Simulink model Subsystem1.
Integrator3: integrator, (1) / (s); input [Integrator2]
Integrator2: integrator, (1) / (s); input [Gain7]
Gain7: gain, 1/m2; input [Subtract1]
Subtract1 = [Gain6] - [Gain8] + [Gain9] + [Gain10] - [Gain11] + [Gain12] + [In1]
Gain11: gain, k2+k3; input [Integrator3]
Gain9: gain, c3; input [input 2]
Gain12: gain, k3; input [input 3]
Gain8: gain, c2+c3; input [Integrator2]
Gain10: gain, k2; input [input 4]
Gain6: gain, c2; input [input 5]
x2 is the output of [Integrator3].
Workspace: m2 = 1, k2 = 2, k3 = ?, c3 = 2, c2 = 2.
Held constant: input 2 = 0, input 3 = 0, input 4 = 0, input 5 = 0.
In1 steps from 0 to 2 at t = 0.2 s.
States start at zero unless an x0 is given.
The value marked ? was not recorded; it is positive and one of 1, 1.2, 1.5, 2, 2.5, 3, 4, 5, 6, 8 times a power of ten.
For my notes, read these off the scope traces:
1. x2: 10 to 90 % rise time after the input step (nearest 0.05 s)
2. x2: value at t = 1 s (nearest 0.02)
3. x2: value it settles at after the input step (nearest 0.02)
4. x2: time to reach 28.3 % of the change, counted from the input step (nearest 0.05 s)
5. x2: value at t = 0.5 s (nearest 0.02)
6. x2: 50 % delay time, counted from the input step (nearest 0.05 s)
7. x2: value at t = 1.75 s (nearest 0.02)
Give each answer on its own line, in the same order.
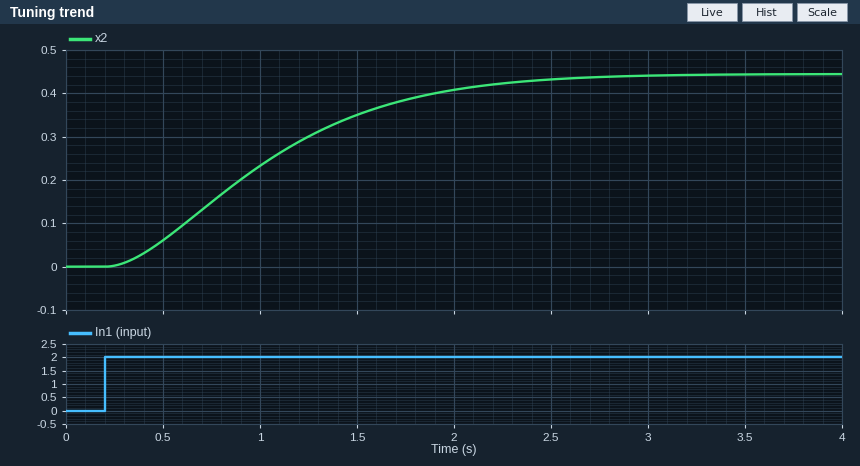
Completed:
1.45 s
0.24
0.44
0.50 s
0.06
0.75 s
0.38
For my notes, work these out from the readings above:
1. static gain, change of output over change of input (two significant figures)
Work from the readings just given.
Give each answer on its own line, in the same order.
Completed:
0.22
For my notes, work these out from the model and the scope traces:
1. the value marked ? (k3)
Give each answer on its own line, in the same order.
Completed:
2.5
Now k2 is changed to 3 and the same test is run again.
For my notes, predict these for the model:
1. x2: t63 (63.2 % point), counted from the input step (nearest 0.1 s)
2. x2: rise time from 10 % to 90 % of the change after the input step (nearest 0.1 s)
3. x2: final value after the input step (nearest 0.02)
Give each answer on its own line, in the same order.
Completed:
0.8 s
1.1 s
0.36
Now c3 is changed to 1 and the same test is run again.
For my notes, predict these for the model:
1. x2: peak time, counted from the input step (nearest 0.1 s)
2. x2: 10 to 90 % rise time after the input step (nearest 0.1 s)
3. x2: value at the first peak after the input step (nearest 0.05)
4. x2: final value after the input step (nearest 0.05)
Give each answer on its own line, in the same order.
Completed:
2.1 s
1.0 s
0.45
0.45
